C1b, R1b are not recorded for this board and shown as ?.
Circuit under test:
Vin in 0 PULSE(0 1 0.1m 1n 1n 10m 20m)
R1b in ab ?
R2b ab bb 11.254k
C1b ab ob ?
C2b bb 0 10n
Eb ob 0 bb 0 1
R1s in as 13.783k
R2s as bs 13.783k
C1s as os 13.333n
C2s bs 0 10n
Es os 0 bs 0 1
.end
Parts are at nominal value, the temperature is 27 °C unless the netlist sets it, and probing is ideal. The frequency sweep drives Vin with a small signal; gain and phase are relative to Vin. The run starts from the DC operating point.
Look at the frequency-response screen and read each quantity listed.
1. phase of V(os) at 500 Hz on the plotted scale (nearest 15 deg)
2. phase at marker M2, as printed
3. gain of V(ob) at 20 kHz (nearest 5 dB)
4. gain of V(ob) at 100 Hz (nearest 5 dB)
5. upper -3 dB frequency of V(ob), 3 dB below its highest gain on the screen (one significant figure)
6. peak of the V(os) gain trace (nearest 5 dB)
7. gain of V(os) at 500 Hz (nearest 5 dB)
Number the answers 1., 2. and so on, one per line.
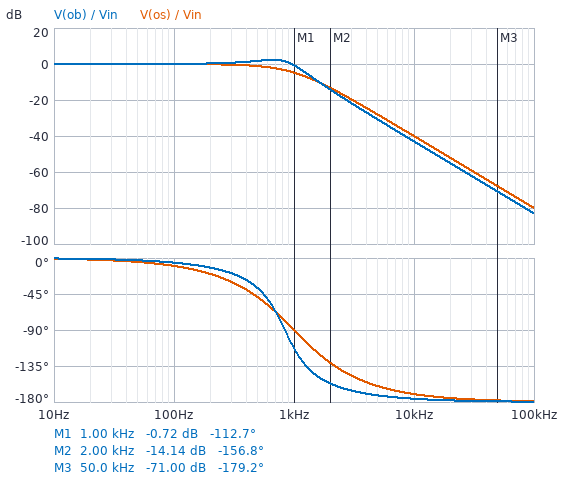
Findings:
1. -45 deg
2. -156.8 deg
3. -55 dB
4. 0 dB
5. 1 kHz
6. 0 dB
7. 0 dB
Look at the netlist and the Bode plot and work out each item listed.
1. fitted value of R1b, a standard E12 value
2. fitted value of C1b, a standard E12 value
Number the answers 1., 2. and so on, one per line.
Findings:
1. 4.7 kΩ
2. 68 nF
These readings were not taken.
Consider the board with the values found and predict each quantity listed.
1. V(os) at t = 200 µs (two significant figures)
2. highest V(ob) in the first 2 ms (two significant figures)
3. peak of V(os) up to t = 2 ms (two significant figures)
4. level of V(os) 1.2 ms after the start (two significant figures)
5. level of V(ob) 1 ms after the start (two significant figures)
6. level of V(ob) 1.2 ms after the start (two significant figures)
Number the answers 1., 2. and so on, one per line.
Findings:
1. 140 mV
2. 1.2 V
3. 1.0 V
4. 1.0 V
5. 1.1 V
6. 990 mV
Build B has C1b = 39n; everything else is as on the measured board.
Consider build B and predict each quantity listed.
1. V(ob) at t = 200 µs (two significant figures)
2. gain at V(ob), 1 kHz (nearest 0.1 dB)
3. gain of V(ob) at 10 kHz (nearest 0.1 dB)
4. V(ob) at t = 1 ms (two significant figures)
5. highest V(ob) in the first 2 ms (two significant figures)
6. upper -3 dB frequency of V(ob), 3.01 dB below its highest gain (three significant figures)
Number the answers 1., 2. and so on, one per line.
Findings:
1. 180 mV
2. -0.2 dB
3. -38.2 dB
4. 1.0 V
5. 1.1 V
6. 1.27 kHz
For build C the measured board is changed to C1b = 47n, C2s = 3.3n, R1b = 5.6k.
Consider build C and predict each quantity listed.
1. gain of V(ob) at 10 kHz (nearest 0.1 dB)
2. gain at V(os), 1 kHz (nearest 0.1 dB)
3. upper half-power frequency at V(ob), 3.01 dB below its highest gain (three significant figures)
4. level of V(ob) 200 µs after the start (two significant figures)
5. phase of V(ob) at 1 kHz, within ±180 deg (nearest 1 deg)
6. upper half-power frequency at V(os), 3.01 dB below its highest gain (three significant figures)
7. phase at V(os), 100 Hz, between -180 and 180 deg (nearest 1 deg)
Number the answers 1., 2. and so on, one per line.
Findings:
1. -41.3 dB
2. 1.1 dB
3. 1.08 kHz
4. 140 mV
5. -99 deg
6. 2.04 kHz
7. -3 deg
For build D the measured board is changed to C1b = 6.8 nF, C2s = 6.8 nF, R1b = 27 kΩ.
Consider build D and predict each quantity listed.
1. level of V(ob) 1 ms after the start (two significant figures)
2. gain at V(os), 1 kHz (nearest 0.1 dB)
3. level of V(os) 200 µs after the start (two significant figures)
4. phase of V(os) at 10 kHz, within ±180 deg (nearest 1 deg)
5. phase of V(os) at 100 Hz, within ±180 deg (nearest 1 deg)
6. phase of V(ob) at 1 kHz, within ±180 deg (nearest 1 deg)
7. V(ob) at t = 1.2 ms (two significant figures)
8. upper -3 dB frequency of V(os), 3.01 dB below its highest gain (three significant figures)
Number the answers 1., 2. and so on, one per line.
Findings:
1. 930 mV
2. -1.7 dB
3. 200 mV
4. -170 deg
5. -7 deg
6. -86 deg
7. 960 mV
8. 1.20 kHz
